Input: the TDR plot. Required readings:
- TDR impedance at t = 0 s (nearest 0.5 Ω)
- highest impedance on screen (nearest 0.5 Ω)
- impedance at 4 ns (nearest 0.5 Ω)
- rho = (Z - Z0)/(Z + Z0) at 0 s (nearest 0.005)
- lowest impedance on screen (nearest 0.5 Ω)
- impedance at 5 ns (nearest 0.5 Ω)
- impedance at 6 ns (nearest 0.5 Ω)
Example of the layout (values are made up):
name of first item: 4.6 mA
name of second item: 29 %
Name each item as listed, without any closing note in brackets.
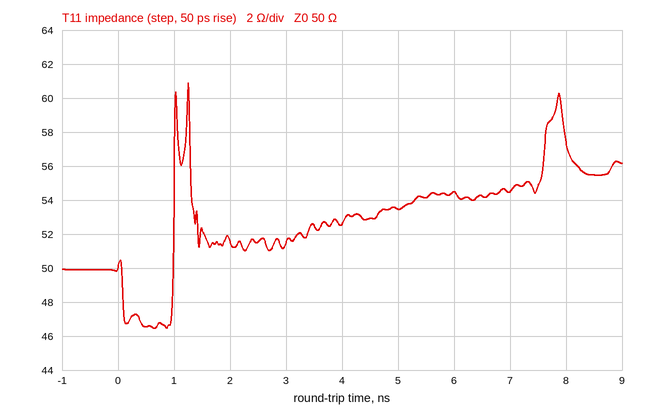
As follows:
TDR impedance at t = 0 s: 50.0 Ω
highest impedance on screen: 61.0 Ω
impedance at 4 ns: 52.5 Ω
rho = (Z - Z0)/(Z + Z0) at 0 s: 0.000
lowest impedance on screen: 46.5 Ω
impedance at 5 ns: 53.5 Ω
impedance at 6 ns: 54.5 Ω
